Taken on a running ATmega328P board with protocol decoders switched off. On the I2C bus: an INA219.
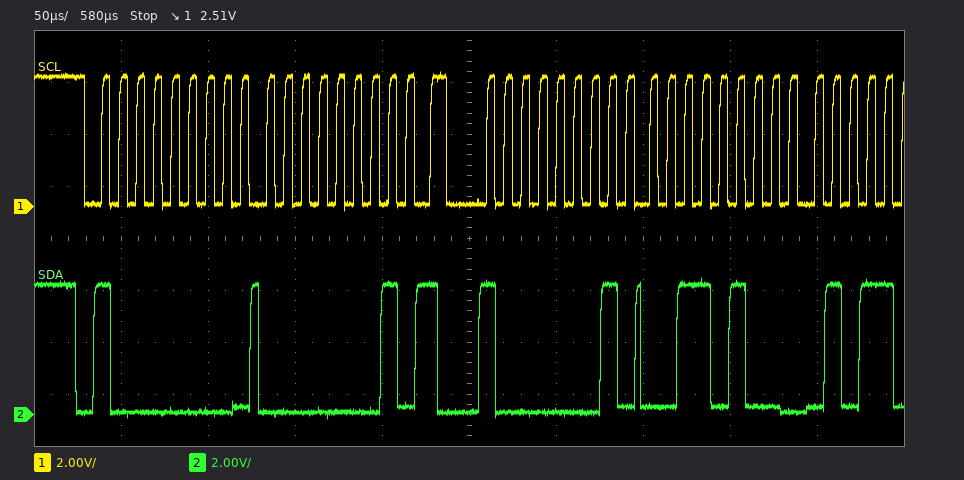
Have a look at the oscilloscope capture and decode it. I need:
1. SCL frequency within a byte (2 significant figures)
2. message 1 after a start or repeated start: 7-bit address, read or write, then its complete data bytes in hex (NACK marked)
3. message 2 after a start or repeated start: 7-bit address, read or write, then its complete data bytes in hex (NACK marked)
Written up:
100 kHz
0x40 write: 01
0x40 read: 34
